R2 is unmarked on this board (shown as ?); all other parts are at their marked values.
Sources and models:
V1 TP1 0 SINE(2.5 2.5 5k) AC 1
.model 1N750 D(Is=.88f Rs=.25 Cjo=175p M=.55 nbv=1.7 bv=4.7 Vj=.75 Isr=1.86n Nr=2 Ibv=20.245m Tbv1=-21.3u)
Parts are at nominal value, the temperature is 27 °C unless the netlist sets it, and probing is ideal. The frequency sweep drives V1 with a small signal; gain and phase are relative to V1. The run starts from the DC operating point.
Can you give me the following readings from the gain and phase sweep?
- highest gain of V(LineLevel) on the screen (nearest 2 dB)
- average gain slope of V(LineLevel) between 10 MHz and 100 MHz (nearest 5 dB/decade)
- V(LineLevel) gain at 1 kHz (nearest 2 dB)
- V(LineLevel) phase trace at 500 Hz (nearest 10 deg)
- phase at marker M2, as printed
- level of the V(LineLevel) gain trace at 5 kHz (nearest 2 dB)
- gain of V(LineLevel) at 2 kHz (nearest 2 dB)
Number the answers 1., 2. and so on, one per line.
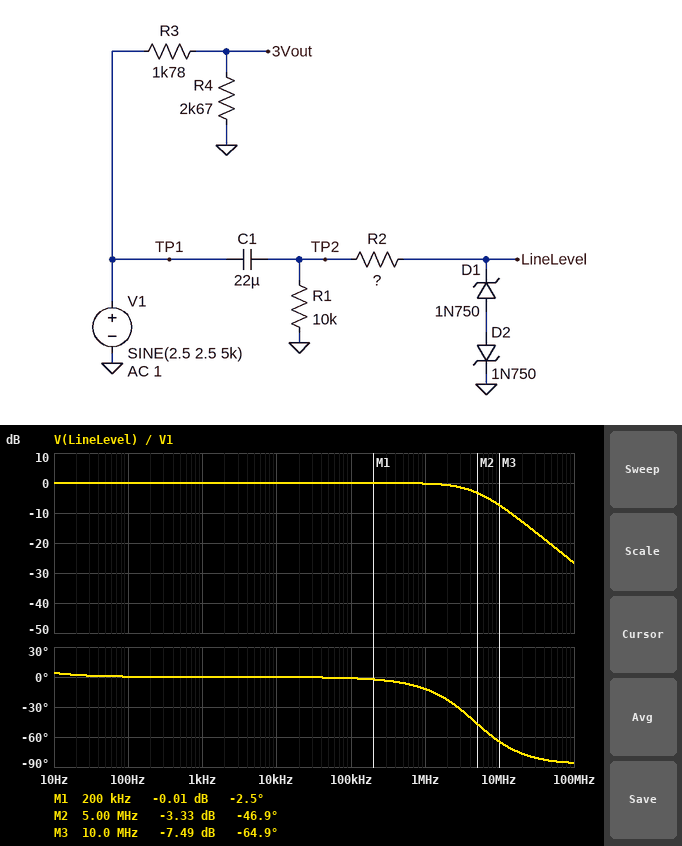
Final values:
1. 0 dB
2. -20 dB/decade
3. 0 dB
4. 0 deg
5. -46.9 deg
6. 0 dB
7. 0 dB
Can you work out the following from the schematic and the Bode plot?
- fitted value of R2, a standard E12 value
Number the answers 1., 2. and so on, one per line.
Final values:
1. 390 Ω
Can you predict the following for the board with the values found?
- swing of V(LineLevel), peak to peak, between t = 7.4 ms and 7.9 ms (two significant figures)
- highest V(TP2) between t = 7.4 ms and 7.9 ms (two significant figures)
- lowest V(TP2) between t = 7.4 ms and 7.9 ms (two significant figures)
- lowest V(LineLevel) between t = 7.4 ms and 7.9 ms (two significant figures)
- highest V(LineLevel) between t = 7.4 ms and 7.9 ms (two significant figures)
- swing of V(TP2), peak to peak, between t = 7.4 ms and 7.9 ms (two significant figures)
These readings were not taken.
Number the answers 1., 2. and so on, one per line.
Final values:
1. 5.0 V
2. 2.5 V
3. -2.5 V
4. -2.5 V
5. 2.5 V
6. 5.0 V
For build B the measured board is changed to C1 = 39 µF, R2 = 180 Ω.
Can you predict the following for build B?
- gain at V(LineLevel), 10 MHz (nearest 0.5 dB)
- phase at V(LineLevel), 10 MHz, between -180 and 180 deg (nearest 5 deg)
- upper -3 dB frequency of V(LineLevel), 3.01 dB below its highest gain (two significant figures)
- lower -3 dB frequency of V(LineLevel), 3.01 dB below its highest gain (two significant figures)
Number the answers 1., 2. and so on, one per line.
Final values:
1. -3.0 dB
2. -45 deg
3. 10 MHz
4. 410 mHz
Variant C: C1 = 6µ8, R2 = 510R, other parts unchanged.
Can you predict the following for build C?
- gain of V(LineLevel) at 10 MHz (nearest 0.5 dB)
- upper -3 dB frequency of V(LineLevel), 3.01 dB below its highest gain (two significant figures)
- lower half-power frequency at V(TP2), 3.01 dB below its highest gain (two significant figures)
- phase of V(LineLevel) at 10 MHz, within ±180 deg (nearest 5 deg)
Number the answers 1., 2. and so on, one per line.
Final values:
1. -9.5 dB
2. 3.6 MHz
3. 2.3 Hz
4. -70 deg
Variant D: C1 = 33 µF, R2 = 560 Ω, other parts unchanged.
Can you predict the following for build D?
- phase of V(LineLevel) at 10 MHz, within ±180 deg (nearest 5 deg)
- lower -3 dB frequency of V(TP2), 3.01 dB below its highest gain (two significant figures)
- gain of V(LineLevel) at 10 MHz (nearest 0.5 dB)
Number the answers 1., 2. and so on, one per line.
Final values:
1. -70 deg
2. 480 mHz
3. -10.0 dB
